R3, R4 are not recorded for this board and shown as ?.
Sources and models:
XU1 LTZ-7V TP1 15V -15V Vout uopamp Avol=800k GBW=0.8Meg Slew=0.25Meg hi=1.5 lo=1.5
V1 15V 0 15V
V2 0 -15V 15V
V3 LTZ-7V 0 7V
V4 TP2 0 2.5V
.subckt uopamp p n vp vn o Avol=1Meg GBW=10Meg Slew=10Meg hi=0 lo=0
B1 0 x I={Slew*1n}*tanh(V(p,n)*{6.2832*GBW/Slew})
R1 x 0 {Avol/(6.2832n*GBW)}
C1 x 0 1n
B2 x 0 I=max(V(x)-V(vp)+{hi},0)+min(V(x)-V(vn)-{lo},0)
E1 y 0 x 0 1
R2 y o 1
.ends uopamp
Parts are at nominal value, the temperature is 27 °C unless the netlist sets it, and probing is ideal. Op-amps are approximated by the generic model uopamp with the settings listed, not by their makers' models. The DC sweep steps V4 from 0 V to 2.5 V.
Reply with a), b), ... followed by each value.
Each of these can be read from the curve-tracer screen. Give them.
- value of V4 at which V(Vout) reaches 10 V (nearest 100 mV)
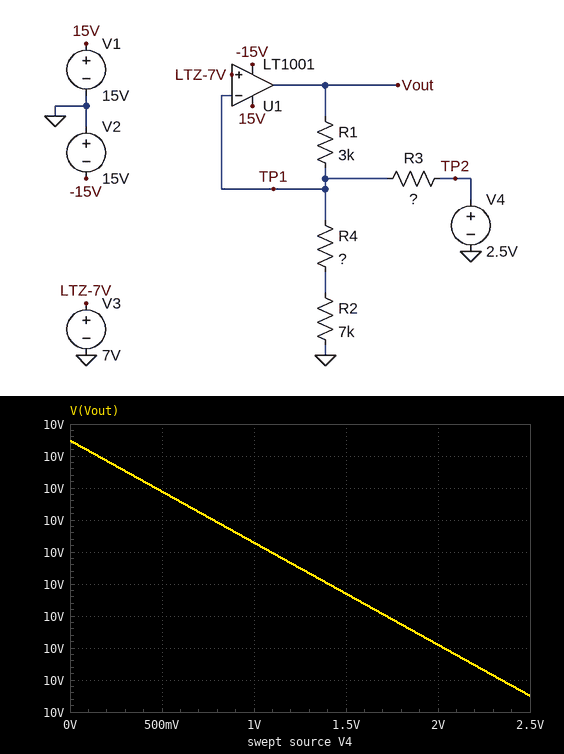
a) 1.4 V
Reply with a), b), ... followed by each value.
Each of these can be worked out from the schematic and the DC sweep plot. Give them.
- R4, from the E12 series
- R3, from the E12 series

a) 18 Ω
b) 470 kΩ
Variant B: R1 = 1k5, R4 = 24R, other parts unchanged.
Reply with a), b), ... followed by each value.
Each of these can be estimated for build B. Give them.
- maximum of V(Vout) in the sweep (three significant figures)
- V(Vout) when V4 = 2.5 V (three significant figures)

a) 8.52 V
b) 8.51 V
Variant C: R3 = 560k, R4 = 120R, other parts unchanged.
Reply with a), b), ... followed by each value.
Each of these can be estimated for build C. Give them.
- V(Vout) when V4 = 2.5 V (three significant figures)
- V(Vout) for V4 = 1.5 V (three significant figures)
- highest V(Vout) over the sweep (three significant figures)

a) 9.97 V
b) 9.98 V
c) 9.99 V
